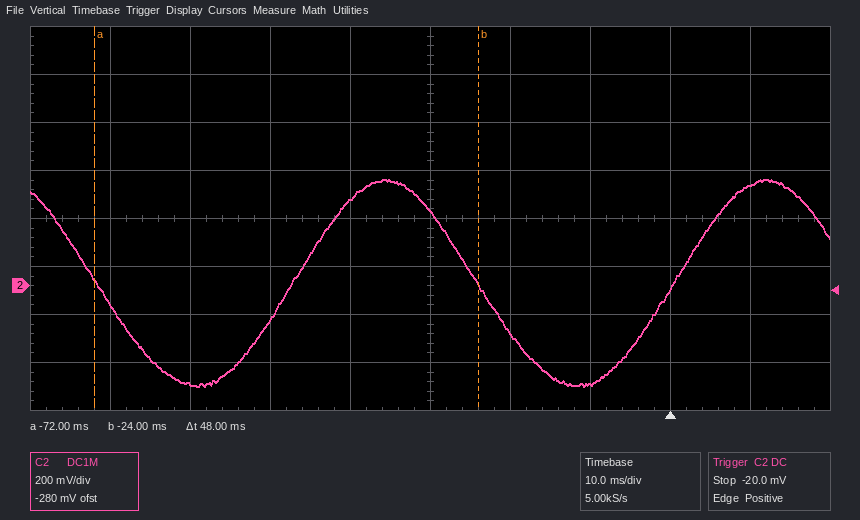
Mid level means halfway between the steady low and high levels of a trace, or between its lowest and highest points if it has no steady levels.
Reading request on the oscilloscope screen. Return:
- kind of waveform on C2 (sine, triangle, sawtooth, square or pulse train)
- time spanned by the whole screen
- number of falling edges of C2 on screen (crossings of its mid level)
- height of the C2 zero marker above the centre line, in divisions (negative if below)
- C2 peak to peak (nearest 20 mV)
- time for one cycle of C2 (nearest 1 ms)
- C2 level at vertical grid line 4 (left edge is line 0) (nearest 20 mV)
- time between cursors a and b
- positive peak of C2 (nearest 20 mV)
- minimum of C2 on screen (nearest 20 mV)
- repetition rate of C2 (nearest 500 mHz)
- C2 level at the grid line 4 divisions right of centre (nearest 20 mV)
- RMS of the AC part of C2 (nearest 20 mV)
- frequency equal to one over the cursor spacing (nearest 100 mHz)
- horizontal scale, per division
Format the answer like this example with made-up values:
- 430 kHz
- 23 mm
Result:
- sine
- 100 ms
- 2
- -1.4 div
- 860 mV
- 48 ms
- 360 mV
- 48 ms
- 440 mV
- -420 mV
- 21.0 Hz
- 420 mV
- 300 mV
- 20.8 Hz
- 10 ms
